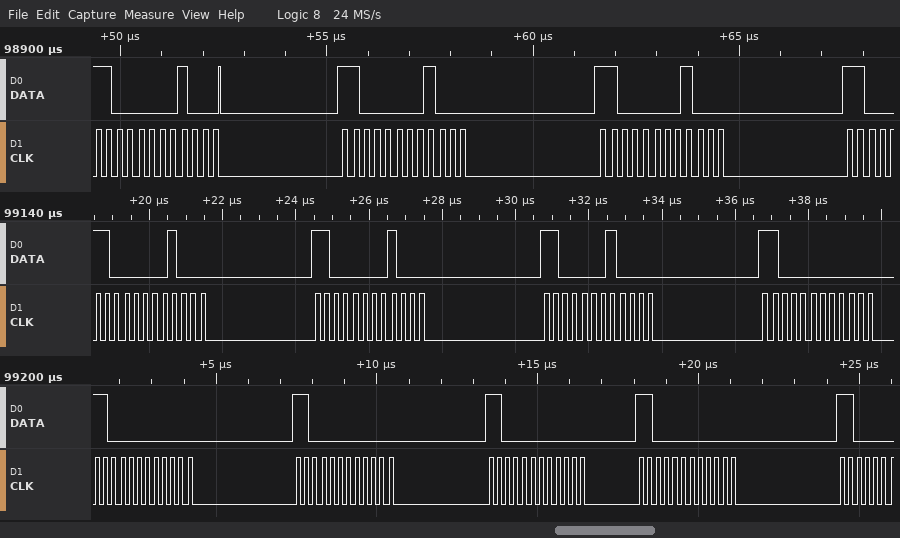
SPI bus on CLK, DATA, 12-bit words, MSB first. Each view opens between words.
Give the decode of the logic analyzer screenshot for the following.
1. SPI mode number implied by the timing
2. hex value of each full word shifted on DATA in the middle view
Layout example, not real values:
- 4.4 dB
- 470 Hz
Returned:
- 0
- C08, C08, C10, C00
